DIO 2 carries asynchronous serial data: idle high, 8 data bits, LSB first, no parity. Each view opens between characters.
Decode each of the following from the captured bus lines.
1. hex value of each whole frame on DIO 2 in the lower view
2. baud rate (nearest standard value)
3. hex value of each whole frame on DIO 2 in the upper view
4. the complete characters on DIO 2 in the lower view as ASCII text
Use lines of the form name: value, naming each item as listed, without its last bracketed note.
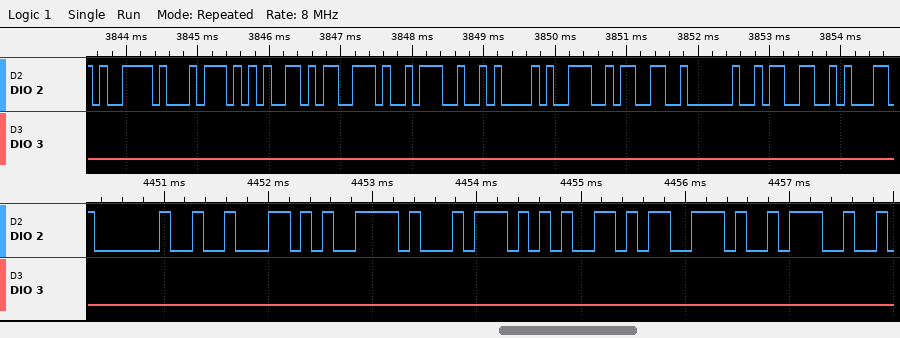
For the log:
hex value of each whole frame on DIO 2 in the lower view: 20, 62, 79, 74, 65, 73, 3A
baud rate: 9600 baud
hex value of each whole frame on DIO 2 in the upper view: 79, 74, 65, 73, 3A, 0A, 39, 33, 20, 33
the complete characters on DIO 2 in the lower view as ASCII text: " bytes:"
